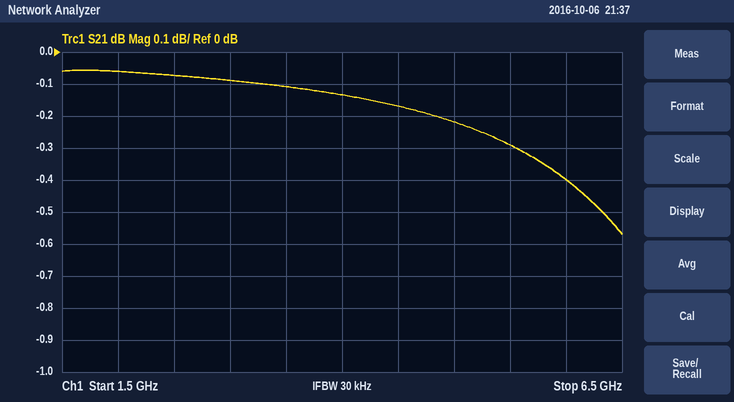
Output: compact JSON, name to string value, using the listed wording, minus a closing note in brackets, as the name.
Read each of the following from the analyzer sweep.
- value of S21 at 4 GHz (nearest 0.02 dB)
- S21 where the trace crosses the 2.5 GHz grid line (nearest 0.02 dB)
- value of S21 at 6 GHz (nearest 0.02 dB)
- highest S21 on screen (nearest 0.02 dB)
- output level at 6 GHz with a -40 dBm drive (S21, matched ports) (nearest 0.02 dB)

{"value of S21 at 4 GHz": "-0.14 dB", "S21 where the trace crosses the 2.5 GHz grid line": "-0.08 dB", "value of S21 at 6 GHz": "-0.40 dB", "highest S21 on screen": "-0.06 dB", "output level at 6 GHz with a -40 dBm drive (S21, matched ports)": "-40.40 dBm"}
